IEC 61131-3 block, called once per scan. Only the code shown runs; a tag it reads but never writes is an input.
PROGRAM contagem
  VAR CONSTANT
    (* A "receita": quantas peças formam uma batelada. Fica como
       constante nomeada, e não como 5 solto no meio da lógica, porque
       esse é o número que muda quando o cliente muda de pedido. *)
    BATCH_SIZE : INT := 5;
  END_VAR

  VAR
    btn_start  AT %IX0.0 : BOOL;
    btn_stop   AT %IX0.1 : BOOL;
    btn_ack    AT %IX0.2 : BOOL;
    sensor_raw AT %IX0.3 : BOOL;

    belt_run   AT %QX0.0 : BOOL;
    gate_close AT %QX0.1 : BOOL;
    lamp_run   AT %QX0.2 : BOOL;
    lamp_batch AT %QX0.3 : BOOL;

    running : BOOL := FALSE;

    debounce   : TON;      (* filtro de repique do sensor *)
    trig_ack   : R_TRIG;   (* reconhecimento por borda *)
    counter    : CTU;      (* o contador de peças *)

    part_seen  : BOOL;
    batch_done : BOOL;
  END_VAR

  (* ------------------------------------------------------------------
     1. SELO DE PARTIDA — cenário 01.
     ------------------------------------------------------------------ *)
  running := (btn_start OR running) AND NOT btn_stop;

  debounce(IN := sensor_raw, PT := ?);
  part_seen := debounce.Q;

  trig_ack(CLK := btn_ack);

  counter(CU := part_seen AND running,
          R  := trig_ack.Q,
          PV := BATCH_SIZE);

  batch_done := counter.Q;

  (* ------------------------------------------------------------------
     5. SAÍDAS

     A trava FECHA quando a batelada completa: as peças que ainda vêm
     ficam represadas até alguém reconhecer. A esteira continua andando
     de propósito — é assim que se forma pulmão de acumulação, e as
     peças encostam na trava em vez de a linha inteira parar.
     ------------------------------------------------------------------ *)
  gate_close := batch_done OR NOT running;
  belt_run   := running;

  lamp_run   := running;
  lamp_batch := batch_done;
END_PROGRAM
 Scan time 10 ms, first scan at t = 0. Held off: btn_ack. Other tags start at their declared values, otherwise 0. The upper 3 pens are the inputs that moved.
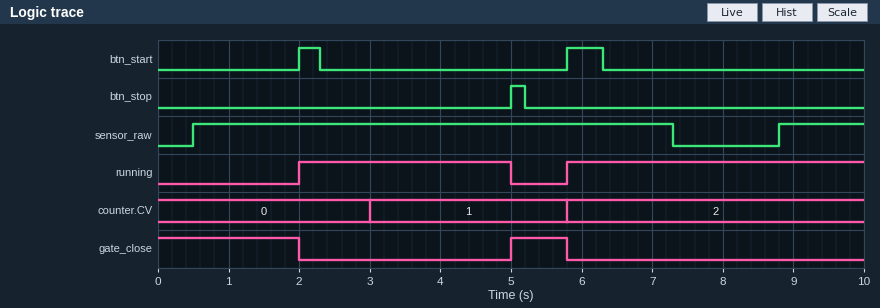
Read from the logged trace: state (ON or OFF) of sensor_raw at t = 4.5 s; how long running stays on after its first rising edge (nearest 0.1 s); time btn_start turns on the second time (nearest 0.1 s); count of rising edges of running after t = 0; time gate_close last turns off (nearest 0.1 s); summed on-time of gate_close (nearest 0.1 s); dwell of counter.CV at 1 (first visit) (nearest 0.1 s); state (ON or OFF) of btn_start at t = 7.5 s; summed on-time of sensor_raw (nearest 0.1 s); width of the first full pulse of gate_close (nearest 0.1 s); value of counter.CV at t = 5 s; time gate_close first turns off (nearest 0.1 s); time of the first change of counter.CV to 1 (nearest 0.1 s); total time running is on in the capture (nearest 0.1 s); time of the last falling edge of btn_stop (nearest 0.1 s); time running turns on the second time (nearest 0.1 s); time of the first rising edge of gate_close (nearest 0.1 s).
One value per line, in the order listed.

ON
3.0 s
5.8 s
2
5.8 s
2.8 s
2.8 s
OFF
8.0 s
0.8 s
1
2.0 s
3.0 s
7.2 s
5.2 s
5.8 s
5.0 s
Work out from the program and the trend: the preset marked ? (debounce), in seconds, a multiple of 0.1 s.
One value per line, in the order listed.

2.5 s
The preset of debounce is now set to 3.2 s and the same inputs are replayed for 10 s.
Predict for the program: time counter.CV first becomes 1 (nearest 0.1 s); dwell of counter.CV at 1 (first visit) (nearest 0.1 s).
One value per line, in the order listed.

3.7 s
2.1 s
